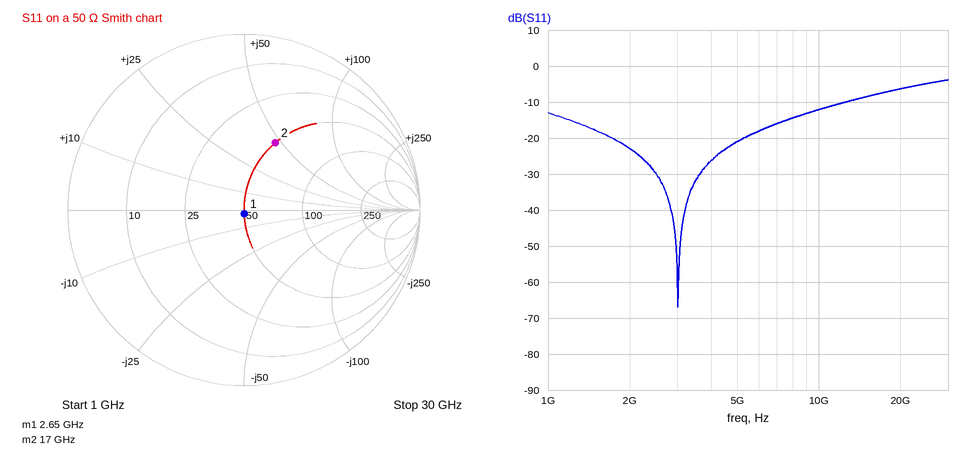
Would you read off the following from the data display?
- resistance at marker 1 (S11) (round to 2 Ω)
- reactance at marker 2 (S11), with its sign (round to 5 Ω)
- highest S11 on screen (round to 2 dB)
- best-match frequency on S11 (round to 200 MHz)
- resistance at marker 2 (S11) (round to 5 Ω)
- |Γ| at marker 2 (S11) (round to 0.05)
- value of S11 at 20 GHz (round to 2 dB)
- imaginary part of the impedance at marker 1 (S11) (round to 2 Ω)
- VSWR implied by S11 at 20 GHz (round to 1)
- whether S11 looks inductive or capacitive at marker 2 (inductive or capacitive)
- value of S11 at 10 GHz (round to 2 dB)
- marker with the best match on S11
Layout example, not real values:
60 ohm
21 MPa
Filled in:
50 Ω
+45 Ω
-4 dB
3.0 GHz
50 Ω
0.40
-6 dB
-2 Ω
3
inductive
-12 dB
marker 1
